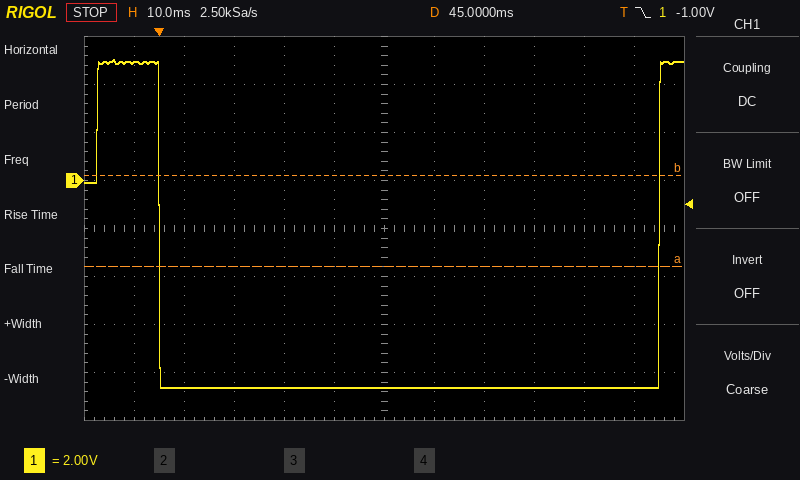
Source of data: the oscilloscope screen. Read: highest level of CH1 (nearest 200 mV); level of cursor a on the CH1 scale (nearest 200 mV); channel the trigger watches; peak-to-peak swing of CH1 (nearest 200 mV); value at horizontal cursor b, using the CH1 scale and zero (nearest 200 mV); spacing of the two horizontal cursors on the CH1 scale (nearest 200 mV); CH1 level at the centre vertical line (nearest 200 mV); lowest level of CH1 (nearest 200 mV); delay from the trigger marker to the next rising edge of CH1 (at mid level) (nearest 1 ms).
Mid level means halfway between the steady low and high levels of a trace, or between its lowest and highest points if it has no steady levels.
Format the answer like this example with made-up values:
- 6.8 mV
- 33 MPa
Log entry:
- 5.0 V
- -3.6 V
- CH1
- 13.6 V
- 200 mV
- 3.8 V
- -8.6 V
- -8.6 V
- 100 ms
